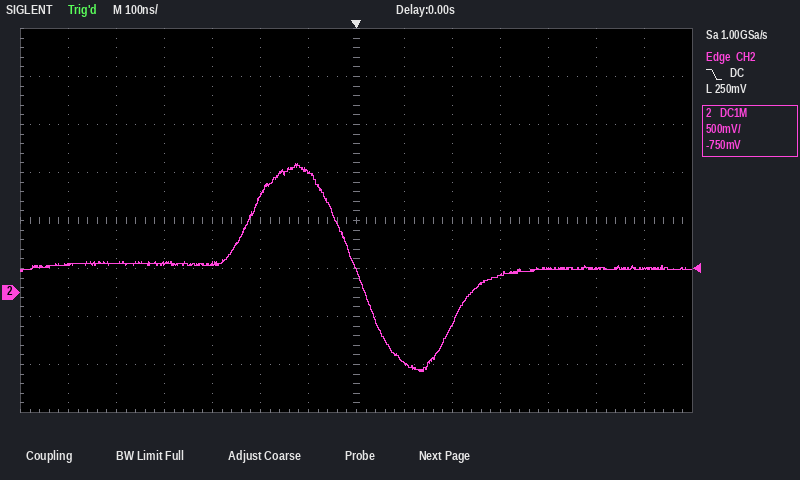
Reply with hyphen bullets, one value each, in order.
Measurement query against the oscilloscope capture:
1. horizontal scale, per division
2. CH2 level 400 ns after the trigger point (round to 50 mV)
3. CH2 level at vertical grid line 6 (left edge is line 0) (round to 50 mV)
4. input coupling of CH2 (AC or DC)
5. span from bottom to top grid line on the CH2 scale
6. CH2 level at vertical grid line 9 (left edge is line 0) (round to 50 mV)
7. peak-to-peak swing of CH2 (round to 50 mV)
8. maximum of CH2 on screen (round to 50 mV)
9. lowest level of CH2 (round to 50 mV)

- 100 ns
- 250 mV
- 1.25 V
- DC
- 4 V
- -350 mV
- 2.15 V
- 1.35 V
- -800 mV
